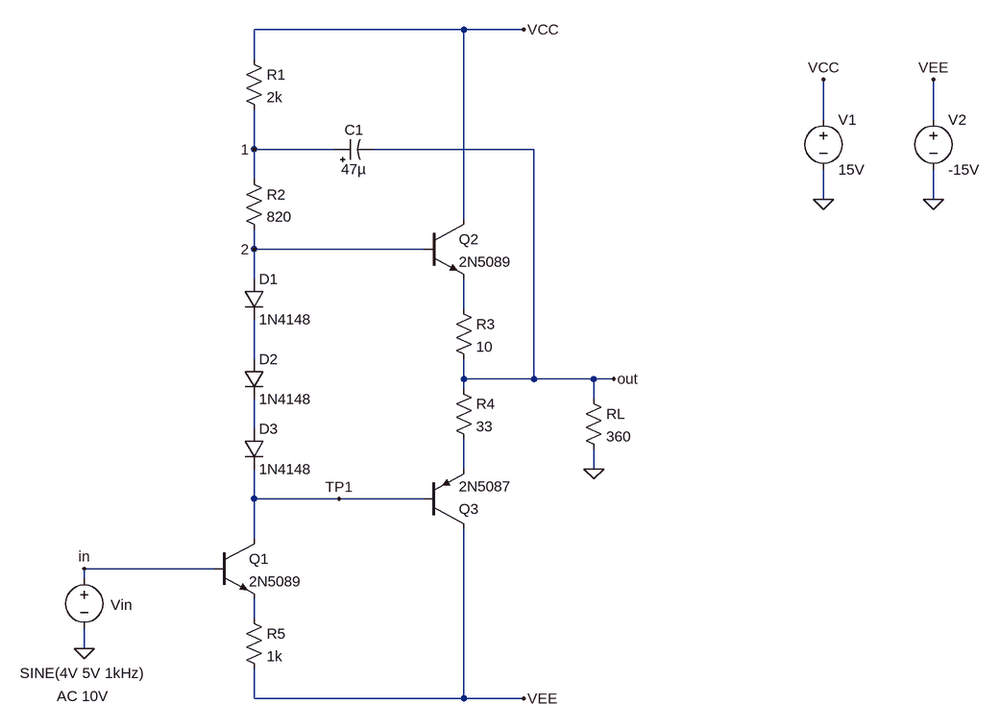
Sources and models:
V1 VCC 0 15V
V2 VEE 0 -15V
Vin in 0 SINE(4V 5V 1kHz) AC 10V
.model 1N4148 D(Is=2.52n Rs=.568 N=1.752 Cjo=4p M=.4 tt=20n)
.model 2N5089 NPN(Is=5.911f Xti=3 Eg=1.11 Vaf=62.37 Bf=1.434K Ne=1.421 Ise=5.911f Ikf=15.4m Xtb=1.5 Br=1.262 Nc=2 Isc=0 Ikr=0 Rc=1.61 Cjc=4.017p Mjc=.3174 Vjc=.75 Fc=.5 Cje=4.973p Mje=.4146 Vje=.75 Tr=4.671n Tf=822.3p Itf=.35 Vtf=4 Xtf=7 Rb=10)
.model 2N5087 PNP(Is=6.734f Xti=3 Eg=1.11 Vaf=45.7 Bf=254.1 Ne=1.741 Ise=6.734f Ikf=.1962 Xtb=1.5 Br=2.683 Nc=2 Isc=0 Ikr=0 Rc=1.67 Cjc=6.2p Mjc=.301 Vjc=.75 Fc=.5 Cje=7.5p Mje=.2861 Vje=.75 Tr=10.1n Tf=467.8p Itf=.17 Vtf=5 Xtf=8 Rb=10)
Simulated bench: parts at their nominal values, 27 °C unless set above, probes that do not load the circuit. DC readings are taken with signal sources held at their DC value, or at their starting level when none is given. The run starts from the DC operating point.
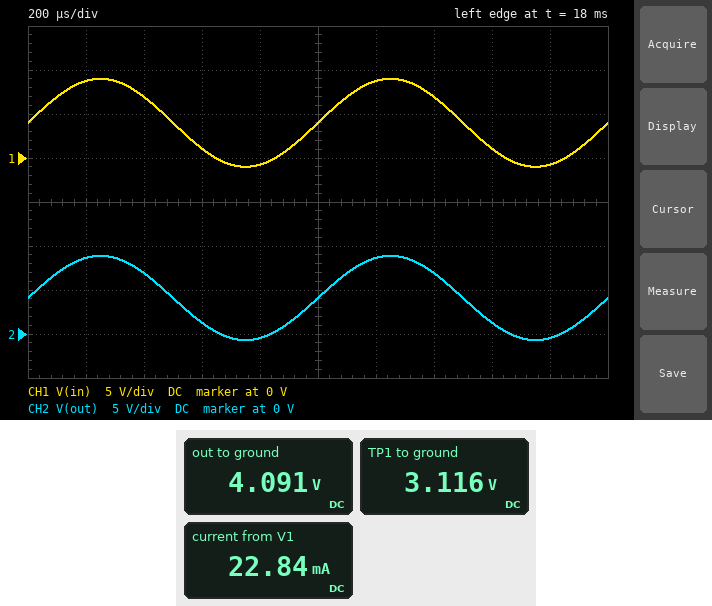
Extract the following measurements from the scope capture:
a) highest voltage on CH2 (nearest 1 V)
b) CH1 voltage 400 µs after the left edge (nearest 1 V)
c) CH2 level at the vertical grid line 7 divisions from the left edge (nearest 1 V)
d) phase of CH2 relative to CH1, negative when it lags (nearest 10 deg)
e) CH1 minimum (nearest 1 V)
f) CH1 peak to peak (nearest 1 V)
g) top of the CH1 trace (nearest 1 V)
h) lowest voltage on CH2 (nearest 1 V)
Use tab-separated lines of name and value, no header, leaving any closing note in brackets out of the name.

highest voltage on CH2	9 V
CH1 voltage 400 µs after the left edge	7 V
CH2 level at the vertical grid line 7 divisions from the left edge	7 V
phase of CH2 relative to CH1, negative when it lags	0 deg
CH1 minimum	-1 V
CH1 peak to peak	10 V
top of the CH1 trace	9 V
lowest voltage on CH2	-1 V
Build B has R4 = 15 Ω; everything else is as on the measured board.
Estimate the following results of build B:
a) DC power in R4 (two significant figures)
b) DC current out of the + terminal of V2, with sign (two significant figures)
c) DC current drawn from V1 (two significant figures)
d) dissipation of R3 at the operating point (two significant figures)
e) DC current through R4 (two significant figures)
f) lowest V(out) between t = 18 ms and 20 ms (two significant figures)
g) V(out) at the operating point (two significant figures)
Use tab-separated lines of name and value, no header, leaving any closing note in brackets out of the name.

DC power in R4	2.5 mW
DC current out of the + terminal of V2, with sign	-31 mA
DC current drawn from V1	28 mA
dissipation of R3 at the operating point	5.8 mW
DC current through R4	13 mA
lowest V(out) between t = 18 ms and 20 ms	-790 mV
V(out) at the operating point	4.0 V
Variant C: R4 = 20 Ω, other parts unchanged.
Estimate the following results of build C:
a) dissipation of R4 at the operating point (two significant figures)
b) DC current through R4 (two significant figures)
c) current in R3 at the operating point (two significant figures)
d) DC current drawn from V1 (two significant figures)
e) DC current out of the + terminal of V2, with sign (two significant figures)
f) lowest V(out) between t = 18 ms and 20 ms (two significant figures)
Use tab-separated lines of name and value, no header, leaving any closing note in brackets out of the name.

dissipation of R4 at the operating point	2.4 mW
DC current through R4	11 mA
current in R3 at the operating point	22 mA
DC current drawn from V1	26 mA
DC current out of the + terminal of V2, with sign	-29 mA
lowest V(out) between t = 18 ms and 20 ms	-750 mV
